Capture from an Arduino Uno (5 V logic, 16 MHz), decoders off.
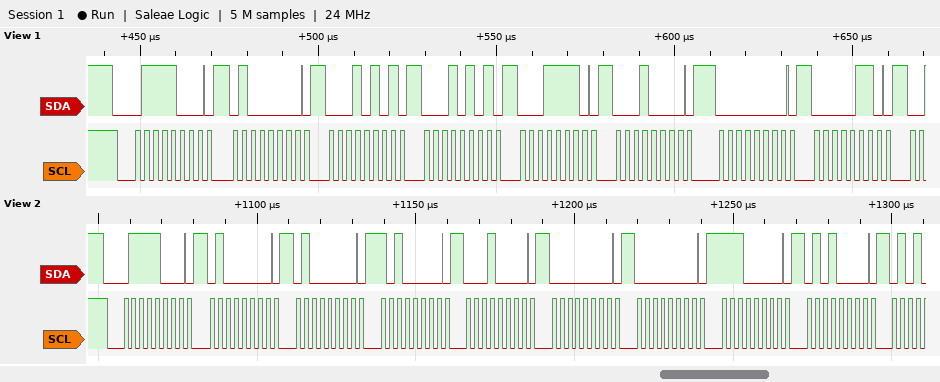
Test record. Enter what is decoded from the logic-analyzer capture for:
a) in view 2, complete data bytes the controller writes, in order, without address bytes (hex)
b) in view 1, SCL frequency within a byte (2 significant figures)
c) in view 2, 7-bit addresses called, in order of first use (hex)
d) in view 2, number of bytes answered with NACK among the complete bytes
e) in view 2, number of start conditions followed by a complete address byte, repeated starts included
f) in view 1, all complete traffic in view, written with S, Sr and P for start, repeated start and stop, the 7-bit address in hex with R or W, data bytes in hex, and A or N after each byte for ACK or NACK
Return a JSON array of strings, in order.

["40 40 A0 10 00 00 E0 50", "400 kHz", "0x3C", "0", "1", "S 3CW A 40 A 15 A 15 A 1E A 10 A 00 A 06 A"]
